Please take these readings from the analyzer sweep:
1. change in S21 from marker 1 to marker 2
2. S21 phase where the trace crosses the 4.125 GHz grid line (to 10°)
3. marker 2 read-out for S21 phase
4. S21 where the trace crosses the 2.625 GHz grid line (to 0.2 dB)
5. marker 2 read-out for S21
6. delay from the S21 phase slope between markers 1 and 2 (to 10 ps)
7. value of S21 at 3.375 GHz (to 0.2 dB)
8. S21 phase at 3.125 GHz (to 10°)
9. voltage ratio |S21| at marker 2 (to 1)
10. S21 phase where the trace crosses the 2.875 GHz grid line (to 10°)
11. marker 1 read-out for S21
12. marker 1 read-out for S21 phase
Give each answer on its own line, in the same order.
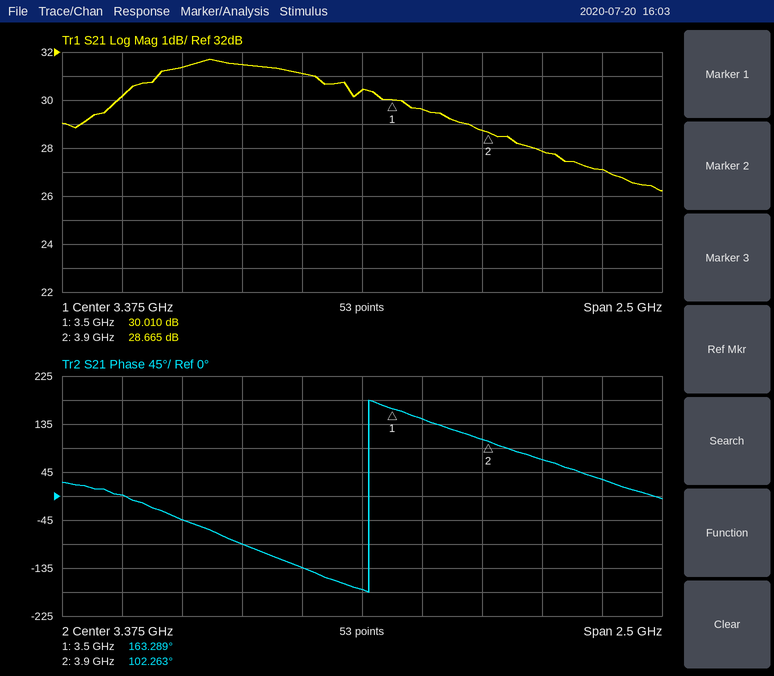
-1.345 dB
70°
102.263°
31.4 dB
28.665 dB
420 ps
30.4 dB
-130°
27
-90°
30.010 dB
163.289°
